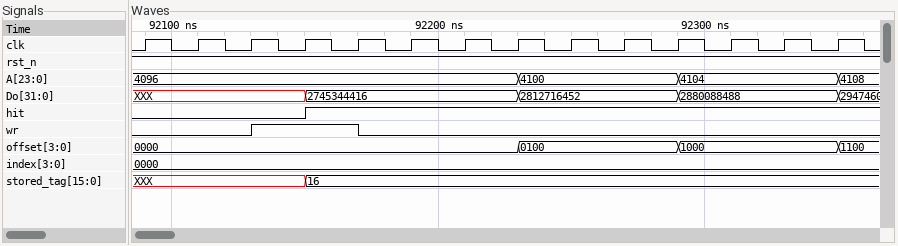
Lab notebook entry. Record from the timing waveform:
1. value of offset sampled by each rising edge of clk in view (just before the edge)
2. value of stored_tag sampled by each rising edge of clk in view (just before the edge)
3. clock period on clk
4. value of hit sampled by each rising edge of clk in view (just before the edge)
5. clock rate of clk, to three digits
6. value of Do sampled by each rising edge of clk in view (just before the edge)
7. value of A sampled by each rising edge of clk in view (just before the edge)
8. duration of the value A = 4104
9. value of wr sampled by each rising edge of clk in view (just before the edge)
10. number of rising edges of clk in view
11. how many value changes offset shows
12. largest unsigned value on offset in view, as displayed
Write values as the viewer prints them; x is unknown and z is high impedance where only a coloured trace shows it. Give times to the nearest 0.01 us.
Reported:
0000, 0000, 0000, 0000, 0000, 0000, 0000, 0000, 0100, 0100, 0100, 1000, 1000, 1000
XXX, XXX, XXX, XXX, 16, 16, 16, 16, 16, 16, 16, 16, 16, 16
0.02 us
0 0 0 0 1 1 1 1 1 1 1 1 1 1
50.0 MHz
XXX, XXX, XXX, XXX, 2745344416, 2745344416, 2745344416, 2745344416, 2812716452, 2812716452, 2812716452, 2880088488, 2880088488, 2880088488
4096, 4096, 4096, 4096, 4096, 4096, 4096, 4096, 4100, 4100, 4100, 4104, 4104, 4104
0.06 us
0 0 0 1 1 0 0 0 0 0 0 0 0 0
14
3
1100
